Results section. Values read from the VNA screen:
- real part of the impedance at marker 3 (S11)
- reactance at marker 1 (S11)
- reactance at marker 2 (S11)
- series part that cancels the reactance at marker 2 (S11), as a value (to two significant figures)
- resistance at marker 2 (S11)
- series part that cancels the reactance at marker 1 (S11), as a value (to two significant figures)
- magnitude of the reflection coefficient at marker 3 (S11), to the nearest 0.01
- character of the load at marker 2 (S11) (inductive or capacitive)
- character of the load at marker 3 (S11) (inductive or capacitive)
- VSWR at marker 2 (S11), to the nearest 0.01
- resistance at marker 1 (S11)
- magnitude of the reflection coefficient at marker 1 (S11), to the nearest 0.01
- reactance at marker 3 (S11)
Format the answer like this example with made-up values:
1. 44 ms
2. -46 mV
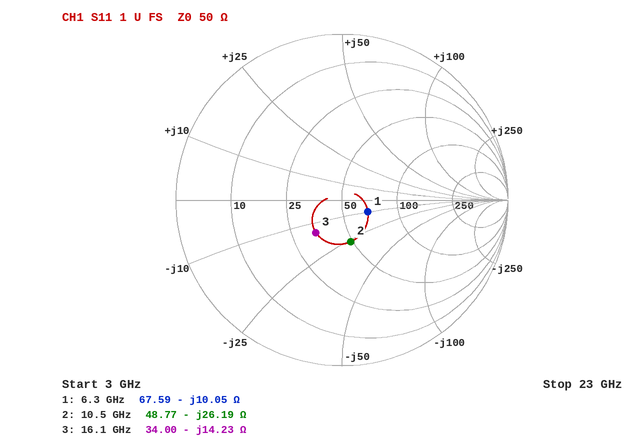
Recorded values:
1. 34.00 Ω
2. -10.05 Ω
3. -26.19 Ω
4. 400 pH
5. 48.77 Ω
6. 250 pH
7. 0.25
8. capacitive
9. capacitive
10. 1.69
11. 67.59 Ω
12. 0.17
13. -14.23 Ω
